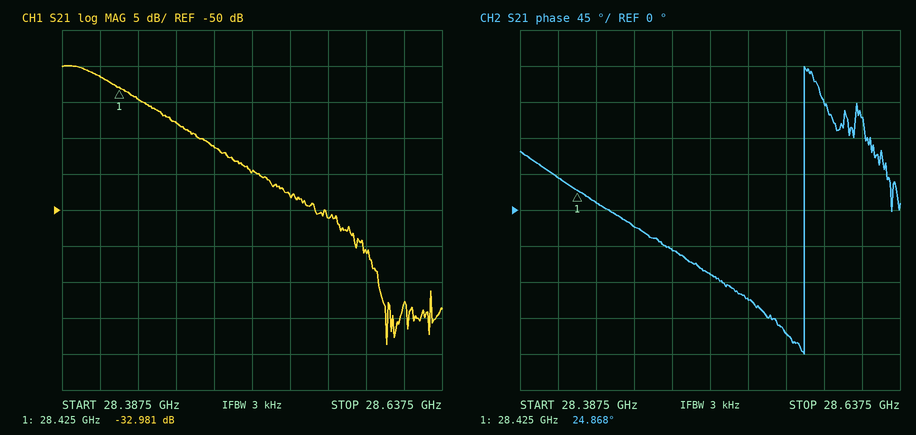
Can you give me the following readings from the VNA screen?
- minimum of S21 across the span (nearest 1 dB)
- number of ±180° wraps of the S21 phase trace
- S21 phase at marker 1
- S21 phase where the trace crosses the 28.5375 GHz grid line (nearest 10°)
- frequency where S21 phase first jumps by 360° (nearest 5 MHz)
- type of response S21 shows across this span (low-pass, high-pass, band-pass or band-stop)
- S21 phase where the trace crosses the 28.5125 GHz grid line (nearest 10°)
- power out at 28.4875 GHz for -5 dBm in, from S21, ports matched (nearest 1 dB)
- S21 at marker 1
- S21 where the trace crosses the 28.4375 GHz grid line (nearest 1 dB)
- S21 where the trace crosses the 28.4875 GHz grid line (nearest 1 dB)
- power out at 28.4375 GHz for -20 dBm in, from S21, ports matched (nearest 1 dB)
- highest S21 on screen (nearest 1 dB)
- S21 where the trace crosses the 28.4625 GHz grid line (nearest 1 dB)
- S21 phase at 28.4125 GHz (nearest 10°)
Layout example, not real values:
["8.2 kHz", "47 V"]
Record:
["-69 dB", "1", "24.868°", "-110°", "28.575 GHz", "low-pass", "-80°", "-46 dBm", "-32.981 dB", "-35 dB", "-41 dB", "-55 dBm", "-30 dB", "-38 dB", "40°"]
